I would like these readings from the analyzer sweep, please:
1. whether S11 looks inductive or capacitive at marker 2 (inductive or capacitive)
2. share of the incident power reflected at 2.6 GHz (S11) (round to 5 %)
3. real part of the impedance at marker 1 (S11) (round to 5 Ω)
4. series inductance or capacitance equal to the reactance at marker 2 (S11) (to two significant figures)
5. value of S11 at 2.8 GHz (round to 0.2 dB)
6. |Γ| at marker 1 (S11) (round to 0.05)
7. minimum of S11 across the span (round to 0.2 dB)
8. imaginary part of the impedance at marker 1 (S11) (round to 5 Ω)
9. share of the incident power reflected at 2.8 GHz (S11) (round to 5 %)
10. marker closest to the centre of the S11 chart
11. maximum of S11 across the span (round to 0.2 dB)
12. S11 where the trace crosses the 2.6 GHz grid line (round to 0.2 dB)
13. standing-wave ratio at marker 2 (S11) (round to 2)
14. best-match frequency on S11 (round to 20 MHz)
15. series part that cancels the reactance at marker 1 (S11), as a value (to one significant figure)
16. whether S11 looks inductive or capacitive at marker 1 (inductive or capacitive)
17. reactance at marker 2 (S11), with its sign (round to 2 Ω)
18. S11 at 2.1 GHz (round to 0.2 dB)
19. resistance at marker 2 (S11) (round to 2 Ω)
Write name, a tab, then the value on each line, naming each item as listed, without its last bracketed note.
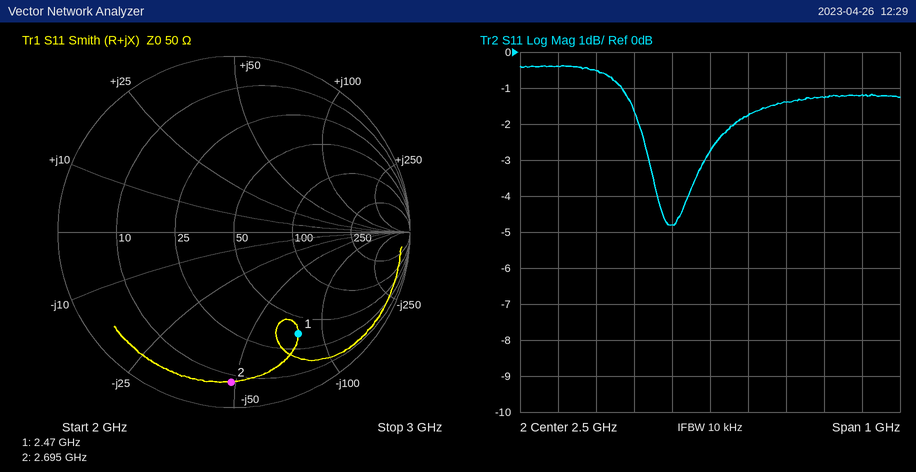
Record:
whether S11 looks inductive or capacitive at marker 2	capacitive
share of the incident power reflected at 2.6 GHz (S11)	65 %
real part of the impedance at marker 1 (S11)	35 Ω
series inductance or capacitance equal to the reactance at marker 2 (S11)	1.2 pF
value of S11 at 2.8 GHz	-1.2 dB
|Γ| at marker 1 (S11)	0.70
minimum of S11 across the span	-4.8 dB
imaginary part of the impedance at marker 1 (S11)	-80 Ω
share of the incident power reflected at 2.8 GHz (S11)	75 %
marker closest to the centre of the S11 chart	marker 1
maximum of S11 across the span	-0.4 dB
S11 where the trace crosses the 2.6 GHz grid line	-1.8 dB
standing-wave ratio at marker 2 (S11)	12
best-match frequency on S11	2.40 GHz
series part that cancels the reactance at marker 1 (S11), as a value	5 nH
whether S11 looks inductive or capacitive at marker 1	capacitive
reactance at marker 2 (S11), with its sign	-48 Ω
S11 at 2.1 GHz	-0.4 dB
resistance at marker 2 (S11)	8 Ω
